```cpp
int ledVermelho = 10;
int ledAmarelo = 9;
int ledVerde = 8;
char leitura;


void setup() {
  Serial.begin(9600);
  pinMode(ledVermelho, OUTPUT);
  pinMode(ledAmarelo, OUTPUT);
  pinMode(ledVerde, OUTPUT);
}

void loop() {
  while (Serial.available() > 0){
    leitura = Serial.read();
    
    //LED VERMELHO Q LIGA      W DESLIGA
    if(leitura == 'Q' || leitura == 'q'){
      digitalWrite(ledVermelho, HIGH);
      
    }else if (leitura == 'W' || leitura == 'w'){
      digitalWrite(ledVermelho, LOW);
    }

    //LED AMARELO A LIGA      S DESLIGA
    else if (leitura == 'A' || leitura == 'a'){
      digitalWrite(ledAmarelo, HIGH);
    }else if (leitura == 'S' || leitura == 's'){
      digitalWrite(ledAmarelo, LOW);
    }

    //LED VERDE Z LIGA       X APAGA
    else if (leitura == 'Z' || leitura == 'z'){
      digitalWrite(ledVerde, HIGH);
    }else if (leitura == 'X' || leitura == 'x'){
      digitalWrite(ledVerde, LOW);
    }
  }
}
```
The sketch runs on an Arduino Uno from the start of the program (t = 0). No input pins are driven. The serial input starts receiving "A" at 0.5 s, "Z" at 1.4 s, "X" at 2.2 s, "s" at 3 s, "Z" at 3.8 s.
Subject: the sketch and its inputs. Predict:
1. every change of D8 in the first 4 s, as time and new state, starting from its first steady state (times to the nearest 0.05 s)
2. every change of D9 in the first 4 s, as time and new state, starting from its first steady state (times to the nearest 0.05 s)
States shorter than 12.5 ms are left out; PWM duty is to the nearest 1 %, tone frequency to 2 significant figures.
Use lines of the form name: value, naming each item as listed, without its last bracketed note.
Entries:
every change of D8 in the first 4 s, as time and new state, starting from its first steady state: 0 s low; 1.4 s high; 2.2 s low; 3.8 s high
every change of D9 in the first 4 s, as time and new state, starting from its first steady state: 0 s low; 0.5 s high; 3 s low
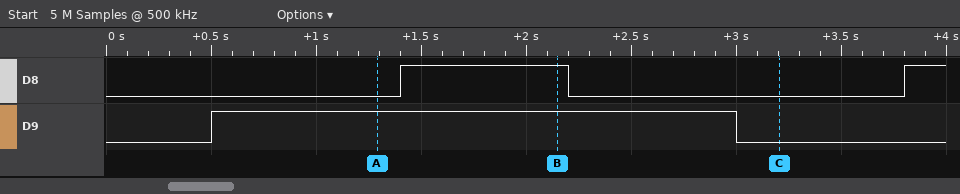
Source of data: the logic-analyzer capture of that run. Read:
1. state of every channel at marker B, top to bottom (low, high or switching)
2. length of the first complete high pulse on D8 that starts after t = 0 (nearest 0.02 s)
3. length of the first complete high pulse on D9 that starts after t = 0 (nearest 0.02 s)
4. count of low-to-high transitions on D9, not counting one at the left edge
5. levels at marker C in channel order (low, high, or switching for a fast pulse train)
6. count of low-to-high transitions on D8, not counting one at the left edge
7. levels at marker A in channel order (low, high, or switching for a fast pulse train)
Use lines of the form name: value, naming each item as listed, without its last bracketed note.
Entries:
state of every channel at marker B, top to bottom: D8 high, D9 high
length of the first complete high pulse on D8 that starts after t = 0: 0.80 s
length of the first complete high pulse on D9 that starts after t = 0: 2.50 s
count of low-to-high transitions on D9, not counting one at the left edge: 1
levels at marker C in channel order: D8 low, D9 low
count of low-to-high transitions on D8, not counting one at the left edge: 2
levels at marker A in channel order: D8 low, D9 high
